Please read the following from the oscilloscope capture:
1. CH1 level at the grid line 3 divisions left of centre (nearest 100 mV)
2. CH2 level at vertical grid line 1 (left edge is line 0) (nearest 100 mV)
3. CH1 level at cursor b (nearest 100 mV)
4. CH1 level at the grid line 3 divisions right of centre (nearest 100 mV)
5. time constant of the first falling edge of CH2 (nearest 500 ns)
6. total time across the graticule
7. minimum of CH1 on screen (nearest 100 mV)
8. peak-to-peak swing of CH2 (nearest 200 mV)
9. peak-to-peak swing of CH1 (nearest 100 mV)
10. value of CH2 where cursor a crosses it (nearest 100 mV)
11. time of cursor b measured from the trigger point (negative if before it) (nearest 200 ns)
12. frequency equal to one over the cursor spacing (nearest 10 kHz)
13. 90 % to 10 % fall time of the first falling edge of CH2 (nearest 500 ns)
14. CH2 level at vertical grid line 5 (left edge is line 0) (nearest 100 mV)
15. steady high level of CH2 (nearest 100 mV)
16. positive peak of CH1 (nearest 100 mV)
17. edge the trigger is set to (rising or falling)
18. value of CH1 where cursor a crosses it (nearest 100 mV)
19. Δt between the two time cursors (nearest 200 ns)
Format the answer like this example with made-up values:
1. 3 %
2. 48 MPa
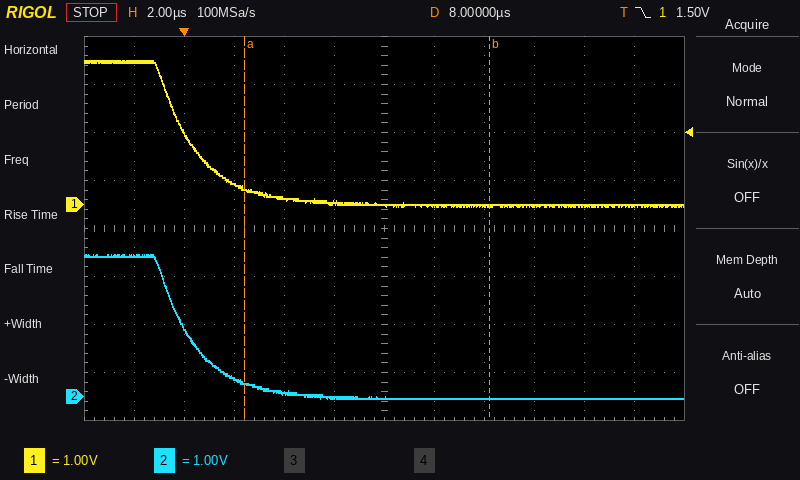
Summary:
1. 400 mV
2. 2.9 V
3. 0.0 V
4. 0.0 V
5. 1.5 µs
6. 24 µs
7. 0.0 V
8. 3.0 V
9. 3.0 V
10. 300 mV
11. +12.2 µs
12. 100 kHz
13. 3.5 µs
14. 0.0 V
15. 2.9 V
16. 3.0 V
17. falling
18. 300 mV
19. 9.8 µs
